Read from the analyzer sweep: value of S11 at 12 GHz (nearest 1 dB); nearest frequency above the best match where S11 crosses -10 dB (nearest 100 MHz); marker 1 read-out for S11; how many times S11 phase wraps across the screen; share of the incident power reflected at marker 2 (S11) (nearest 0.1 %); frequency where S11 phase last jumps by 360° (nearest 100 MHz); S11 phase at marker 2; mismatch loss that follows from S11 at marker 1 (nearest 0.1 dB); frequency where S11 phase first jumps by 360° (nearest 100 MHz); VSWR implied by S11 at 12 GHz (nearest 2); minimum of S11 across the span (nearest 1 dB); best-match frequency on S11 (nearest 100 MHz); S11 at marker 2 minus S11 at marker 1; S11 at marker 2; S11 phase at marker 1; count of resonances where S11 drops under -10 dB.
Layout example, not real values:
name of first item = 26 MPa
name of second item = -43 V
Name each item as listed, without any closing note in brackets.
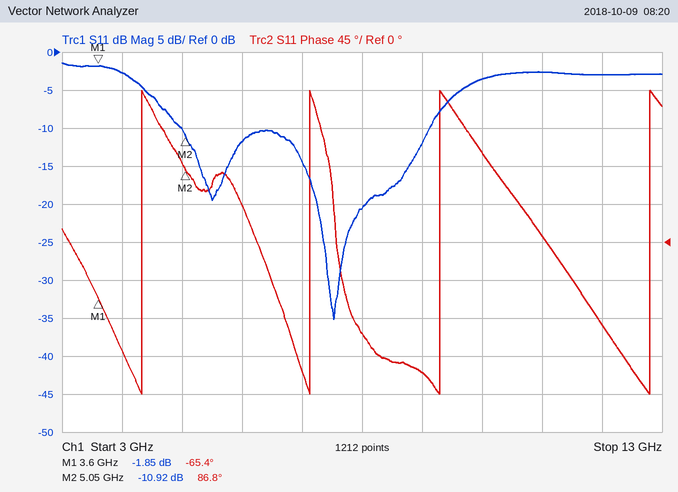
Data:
value of S11 at 12 GHz = -3 dB
nearest frequency above the best match where S11 crosses -10 dB = 9.1 GHz
marker 1 read-out for S11 = -1.85 dB
how many times S11 phase wraps across the screen = 4
share of the incident power reflected at marker 2 (S11) = 8.1 %
frequency where S11 phase last jumps by 360° = 12.8 GHz
S11 phase at marker 2 = 86.8°
mismatch loss that follows from S11 at marker 1 = 4.6 dB
frequency where S11 phase first jumps by 360° = 4.3 GHz
VSWR implied by S11 at 12 GHz = 6
minimum of S11 across the span = -35 dB
best-match frequency on S11 = 7.5 GHz
S11 at marker 2 minus S11 at marker 1 = -9.07 dB
S11 at marker 2 = -10.92 dB
S11 phase at marker 1 = -65.4°
count of resonances where S11 drops under -10 dB = 2
